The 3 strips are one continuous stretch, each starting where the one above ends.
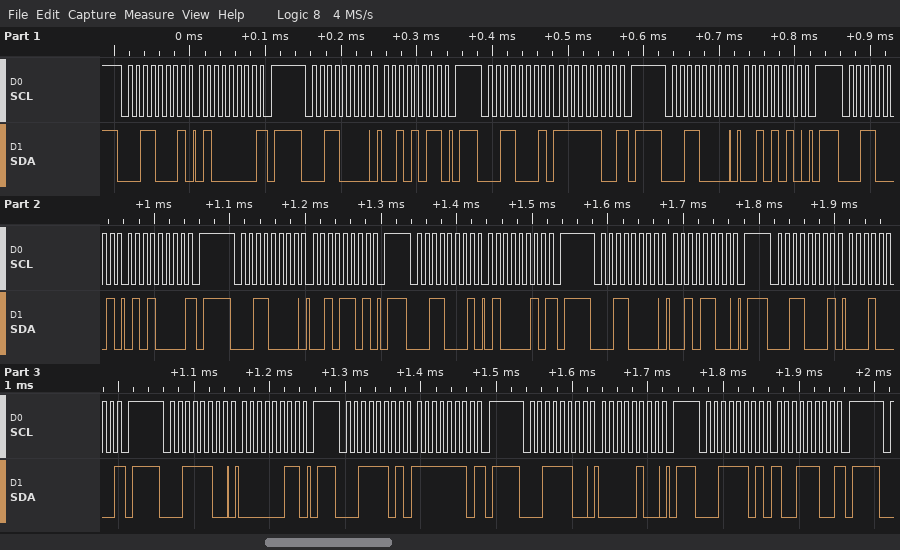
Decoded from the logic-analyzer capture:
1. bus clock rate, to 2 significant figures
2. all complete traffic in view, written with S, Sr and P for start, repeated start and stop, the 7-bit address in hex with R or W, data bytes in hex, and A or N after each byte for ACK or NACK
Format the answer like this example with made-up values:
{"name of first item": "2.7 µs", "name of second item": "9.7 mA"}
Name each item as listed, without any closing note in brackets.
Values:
{"bus clock rate, to 2 significant figures": "100 kHz", "all complete traffic in view, written with S, Sr and P for start, repeated start and stop, the 7-bit address in hex with R or W, data bytes in hex, and A or N after each byte for ACK or NACK": "S 18R A 40 N P S 18W A 2B A P S 18R A FC N P S 18W A 2A A P S 18R A 50 N P S 18W A 2D A P S 18R A 42 N P S 18W A 2C A P S 18R A 10 N P S 1EW A 03 A P S 1ER A FE N P S 1EW A 04 A P S 1ER A 9C N P"}
